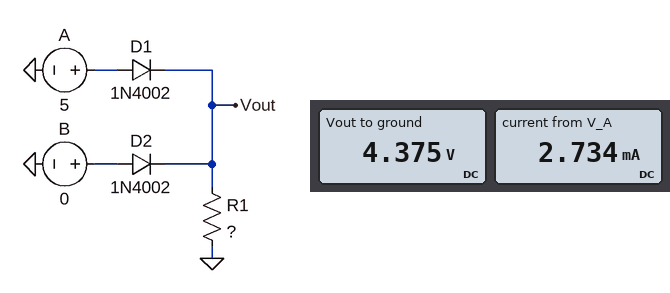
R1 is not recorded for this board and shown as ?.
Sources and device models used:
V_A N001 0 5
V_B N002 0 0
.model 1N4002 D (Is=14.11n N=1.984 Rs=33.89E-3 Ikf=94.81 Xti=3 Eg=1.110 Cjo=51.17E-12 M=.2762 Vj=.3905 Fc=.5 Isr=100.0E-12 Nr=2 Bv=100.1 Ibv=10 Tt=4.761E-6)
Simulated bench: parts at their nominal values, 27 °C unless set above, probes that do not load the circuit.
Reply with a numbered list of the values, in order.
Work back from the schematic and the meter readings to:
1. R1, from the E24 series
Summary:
1. 1.6 kΩ
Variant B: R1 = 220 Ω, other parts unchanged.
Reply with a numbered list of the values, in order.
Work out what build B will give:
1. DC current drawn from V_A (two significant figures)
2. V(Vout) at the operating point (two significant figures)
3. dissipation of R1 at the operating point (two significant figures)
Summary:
1. 19 mA
2. 4.3 V
3. 83 mW
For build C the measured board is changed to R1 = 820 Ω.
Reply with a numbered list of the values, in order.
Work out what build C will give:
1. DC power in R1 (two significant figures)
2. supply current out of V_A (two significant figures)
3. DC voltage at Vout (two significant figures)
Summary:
1. 23 mW
2. 5.3 mA
3. 4.3 V
